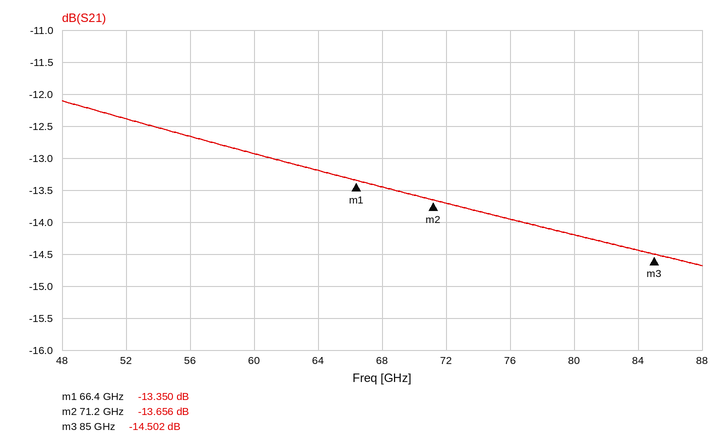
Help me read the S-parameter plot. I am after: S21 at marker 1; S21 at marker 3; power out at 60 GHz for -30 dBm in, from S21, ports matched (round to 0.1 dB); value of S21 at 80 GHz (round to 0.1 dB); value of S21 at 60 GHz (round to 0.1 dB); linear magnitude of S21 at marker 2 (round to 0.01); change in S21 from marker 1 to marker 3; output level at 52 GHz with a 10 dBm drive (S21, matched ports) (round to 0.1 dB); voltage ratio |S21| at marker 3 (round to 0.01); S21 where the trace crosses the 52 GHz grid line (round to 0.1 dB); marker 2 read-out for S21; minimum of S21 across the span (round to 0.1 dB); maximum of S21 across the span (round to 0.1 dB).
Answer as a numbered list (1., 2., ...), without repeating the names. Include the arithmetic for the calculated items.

1. -13.350 dB
2. -14.502 dB
3. -30 dBm + (-12.9 dB) = -42.9 dBm
4. -14.2 dB
5. -12.9 dB
6. 10^(-13.656/20) ≈ 0.21
7. -14.502 − (-13.35) = -1.152 dB
8. 10 dBm + (-12.4 dB) = -2.4 dBm
9. 10^(-14.502/20) ≈ 0.19
10. -12.4 dB
11. -13.656 dB
12. -14.7 dB
13. -12.1 dB
